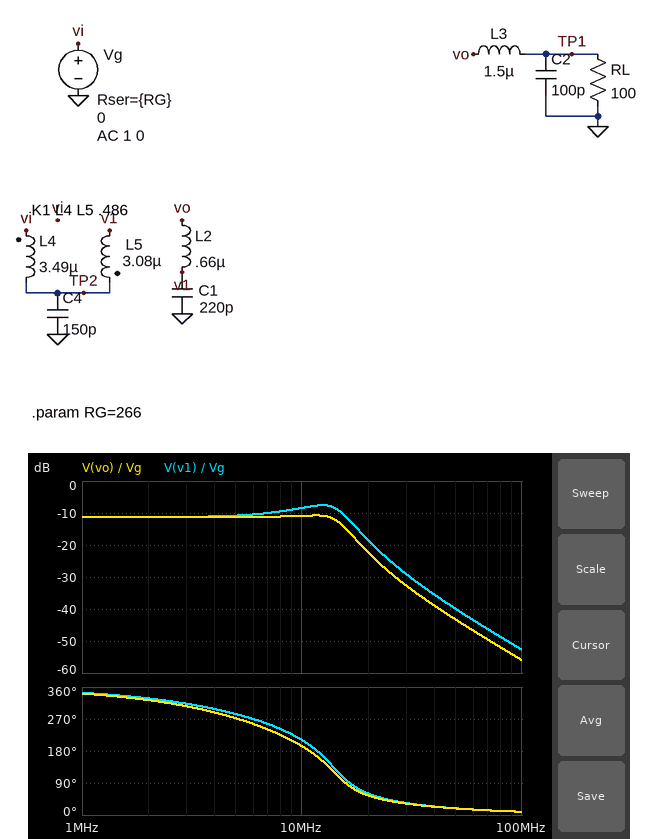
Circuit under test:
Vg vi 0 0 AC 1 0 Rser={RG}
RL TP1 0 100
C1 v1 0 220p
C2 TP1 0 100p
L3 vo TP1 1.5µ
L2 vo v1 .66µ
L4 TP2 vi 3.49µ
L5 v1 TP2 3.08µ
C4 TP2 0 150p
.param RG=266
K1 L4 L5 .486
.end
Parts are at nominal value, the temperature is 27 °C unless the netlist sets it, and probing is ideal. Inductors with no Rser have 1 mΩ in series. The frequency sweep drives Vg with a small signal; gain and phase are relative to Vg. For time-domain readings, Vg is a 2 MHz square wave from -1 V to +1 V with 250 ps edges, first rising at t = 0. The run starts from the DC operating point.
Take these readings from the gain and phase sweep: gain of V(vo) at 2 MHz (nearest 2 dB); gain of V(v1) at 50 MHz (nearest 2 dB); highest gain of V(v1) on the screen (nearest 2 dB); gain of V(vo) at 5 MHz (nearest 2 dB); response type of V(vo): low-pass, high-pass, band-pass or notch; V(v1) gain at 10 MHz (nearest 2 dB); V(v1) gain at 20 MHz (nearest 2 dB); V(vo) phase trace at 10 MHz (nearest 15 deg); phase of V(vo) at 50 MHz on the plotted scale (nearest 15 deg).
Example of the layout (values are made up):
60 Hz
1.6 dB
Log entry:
-12 dB
-40 dB
-8 dB
-12 dB
low-pass
-8 dB
-18 dB
195 deg
15 deg
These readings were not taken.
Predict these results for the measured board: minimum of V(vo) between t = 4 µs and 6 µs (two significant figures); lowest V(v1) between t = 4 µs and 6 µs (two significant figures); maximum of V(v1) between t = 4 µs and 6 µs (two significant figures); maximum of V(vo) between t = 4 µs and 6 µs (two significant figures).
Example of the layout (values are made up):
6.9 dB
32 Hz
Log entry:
-350 mV
-370 mV
370 mV
350 mV
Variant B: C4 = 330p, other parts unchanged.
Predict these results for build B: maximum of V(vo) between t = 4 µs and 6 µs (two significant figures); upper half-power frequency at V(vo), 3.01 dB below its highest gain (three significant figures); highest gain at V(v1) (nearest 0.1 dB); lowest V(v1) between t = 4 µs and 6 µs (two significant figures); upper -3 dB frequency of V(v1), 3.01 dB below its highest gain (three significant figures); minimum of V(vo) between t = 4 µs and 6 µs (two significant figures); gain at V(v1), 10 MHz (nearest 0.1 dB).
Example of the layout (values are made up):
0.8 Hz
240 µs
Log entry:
390 mV
13.2 MHz
-7.2 dB
-420 mV
13.5 MHz
-390 mV
-7.7 dB
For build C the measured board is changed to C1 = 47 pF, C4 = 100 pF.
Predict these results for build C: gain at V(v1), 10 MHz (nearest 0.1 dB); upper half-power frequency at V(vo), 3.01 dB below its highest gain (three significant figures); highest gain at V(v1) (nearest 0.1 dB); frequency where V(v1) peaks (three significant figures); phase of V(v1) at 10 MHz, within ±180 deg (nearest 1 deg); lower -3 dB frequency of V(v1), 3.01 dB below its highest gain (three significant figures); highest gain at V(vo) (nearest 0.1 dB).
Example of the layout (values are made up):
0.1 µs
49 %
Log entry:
-8.2 dB
26.6 MHz
2.6 dB
24.5 MHz
-78 deg
22.0 MHz
-1.2 dB
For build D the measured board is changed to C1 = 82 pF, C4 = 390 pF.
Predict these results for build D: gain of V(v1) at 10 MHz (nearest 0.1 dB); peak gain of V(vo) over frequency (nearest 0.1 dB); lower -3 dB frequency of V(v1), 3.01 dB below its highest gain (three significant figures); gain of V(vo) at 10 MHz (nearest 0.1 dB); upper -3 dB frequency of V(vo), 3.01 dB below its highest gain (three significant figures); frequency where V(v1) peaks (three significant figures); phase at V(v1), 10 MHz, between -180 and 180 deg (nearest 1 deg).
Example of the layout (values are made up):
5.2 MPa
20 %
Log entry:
-11.0 dB
-5.0 dB
15.9 MHz
-13.5 dB
19.5 MHz
17.8 MHz
-144 deg
